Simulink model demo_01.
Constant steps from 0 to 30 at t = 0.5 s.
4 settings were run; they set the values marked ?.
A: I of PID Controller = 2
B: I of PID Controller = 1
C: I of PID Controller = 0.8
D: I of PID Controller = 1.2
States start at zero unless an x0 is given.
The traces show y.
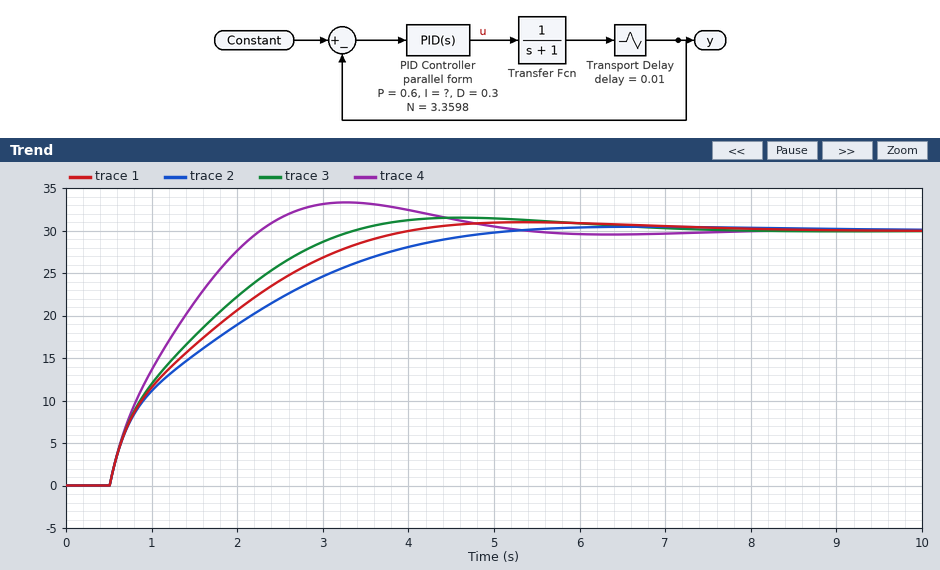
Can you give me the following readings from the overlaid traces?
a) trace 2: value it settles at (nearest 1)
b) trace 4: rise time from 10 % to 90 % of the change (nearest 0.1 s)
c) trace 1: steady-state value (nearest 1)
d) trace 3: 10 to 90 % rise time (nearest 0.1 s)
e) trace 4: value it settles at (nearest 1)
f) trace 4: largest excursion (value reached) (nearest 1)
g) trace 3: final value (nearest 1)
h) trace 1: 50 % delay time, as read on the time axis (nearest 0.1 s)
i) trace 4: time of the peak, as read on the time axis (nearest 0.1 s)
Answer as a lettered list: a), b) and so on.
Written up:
a) 30
b) 1.4 s
c) 30
d) 2.1 s
e) 30
f) 33
g) 30
h) 1.3 s
i) 3.3 s
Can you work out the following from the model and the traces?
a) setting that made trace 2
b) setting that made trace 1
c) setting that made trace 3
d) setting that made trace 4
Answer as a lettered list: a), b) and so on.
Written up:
a) C
b) B
c) D
d) A
